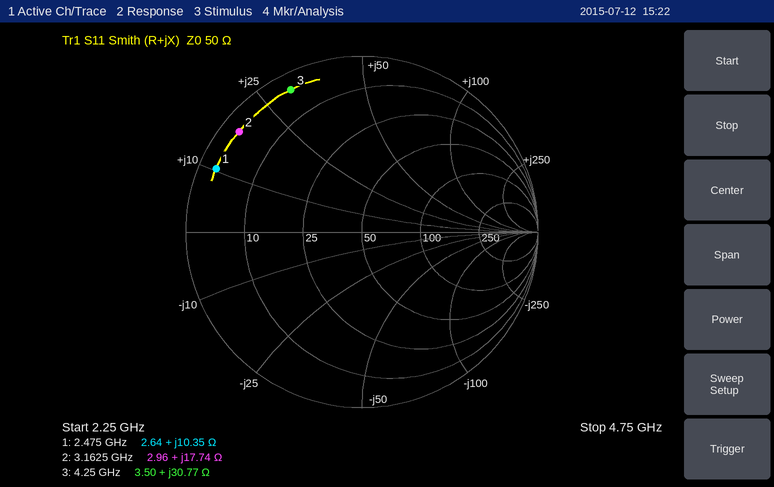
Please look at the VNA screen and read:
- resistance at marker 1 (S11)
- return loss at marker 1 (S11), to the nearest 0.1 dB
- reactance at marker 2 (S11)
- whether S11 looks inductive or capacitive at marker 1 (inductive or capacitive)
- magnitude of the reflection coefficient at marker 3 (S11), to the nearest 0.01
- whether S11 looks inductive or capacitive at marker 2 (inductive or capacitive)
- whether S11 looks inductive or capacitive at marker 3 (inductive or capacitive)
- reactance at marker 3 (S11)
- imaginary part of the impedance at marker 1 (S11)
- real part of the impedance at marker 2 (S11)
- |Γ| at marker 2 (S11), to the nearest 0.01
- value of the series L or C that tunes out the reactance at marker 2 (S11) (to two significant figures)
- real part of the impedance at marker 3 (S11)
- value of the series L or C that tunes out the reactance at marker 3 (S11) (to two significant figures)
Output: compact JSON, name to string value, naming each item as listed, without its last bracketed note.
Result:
{"resistance at marker 1": "2.64 Ω", "return loss at marker 1 (S11), to the nearest 0.1 dB": "0.9 dB", "reactance at marker 2": "+17.74 Ω", "whether S11 looks inductive or capacitive at marker 1": "inductive", "magnitude of the reflection coefficient at marker 3 (S11), to the nearest 0.01": "0.90", "whether S11 looks inductive or capacitive at marker 2": "inductive", "whether S11 looks inductive or capacitive at marker 3": "inductive", "reactance at marker 3": "+30.77 Ω", "imaginary part of the impedance at marker 1": "+10.35 Ω", "real part of the impedance at marker 2": "2.96 Ω", "|Γ| at marker 2 (S11), to the nearest 0.01": "0.90", "value of the series L or C that tunes out the reactance at marker 2 (S11)": "2.8 pF", "real part of the impedance at marker 3": "3.50 Ω", "value of the series L or C that tunes out the reactance at marker 3 (S11)": "1.2 pF"}
